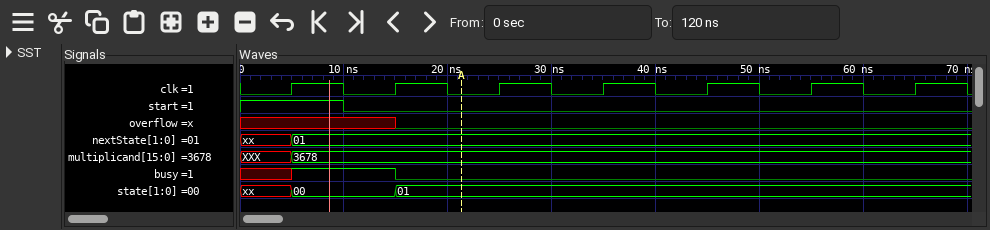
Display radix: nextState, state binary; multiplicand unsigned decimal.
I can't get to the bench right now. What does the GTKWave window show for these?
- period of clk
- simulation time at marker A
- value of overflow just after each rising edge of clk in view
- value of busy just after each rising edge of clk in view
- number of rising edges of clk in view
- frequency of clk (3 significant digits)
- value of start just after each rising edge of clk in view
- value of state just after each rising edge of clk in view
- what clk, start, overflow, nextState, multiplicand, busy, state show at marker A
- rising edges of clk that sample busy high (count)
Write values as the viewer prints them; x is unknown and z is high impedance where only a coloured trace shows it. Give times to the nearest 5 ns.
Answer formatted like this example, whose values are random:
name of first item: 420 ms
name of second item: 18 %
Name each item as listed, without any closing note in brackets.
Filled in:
period of clk: 10 ns
simulation time at marker A: 20 ns
value of overflow just after each rising edge of clk in view: x 0 0 0 0 0 0
value of busy just after each rising edge of clk in view: 1 0 0 0 0 0 0
number of rising edges of clk in view: 7
frequency of clk: 100 MHz
value of start just after each rising edge of clk in view: 1 0 0 0 0 0 0
value of state just after each rising edge of clk in view: 00, 01, 01, 01, 01, 01, 01
what clk, start, overflow, nextState, multiplicand, busy, state show at marker A: clk=0, start=0, overflow=0, nextState=01, multiplicand=3678, busy=0, state=01
rising edges of clk that sample busy high: 1
